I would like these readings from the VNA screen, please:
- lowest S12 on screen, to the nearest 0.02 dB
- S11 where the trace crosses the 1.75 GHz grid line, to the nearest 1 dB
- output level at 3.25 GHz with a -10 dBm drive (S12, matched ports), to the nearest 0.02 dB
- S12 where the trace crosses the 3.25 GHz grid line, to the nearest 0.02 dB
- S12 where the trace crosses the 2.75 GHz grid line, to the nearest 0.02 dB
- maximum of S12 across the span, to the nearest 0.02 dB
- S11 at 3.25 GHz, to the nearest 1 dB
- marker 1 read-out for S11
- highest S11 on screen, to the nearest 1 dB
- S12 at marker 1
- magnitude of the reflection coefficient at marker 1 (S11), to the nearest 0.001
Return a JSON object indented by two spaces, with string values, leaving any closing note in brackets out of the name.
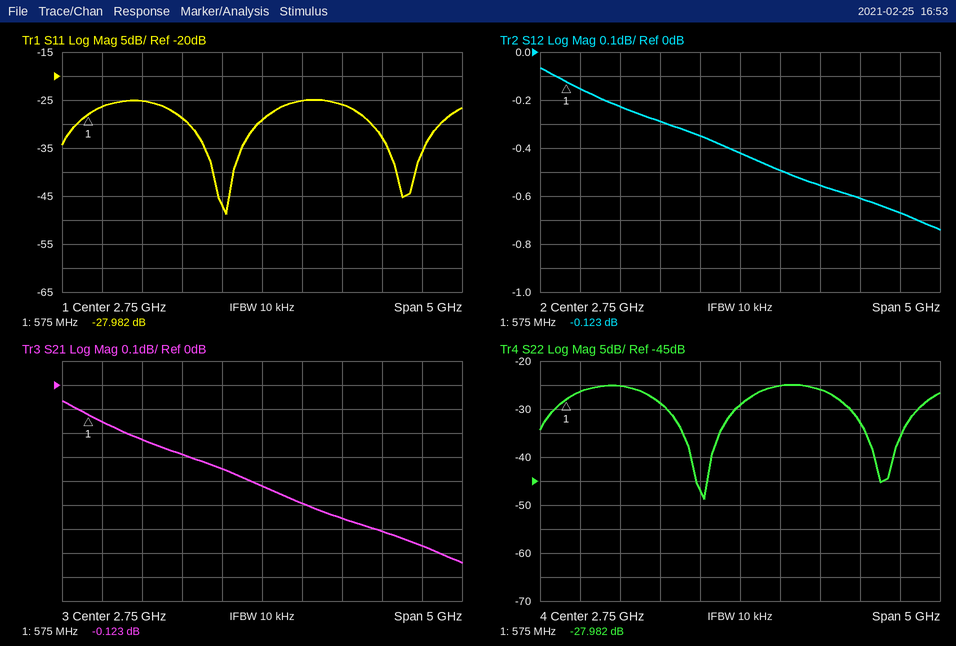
{
  "lowest S12 on screen, to the nearest 0.02 dB": "-0.74 dB",
  "S11 where the trace crosses the 1.75 GHz grid line, to the nearest 1 dB": "-29 dB",
  "output level at 3.25 GHz with a -10 dBm drive (S12, matched ports), to the nearest 0.02 dB": "-10.50 dBm",
  "S12 where the trace crosses the 3.25 GHz grid line, to the nearest 0.02 dB": "-0.50 dB",
  "S12 where the trace crosses the 2.75 GHz grid line, to the nearest 0.02 dB": "-0.42 dB",
  "maximum of S12 across the span, to the nearest 0.02 dB": "-0.06 dB",
  "S11 at 3.25 GHz, to the nearest 1 dB": "-25 dB",
  "marker 1 read-out for S11": "-27.982 dB",
  "highest S11 on screen, to the nearest 1 dB": "-25 dB",
  "S12 at marker 1": "-0.123 dB",
  "magnitude of the reflection coefficient at marker 1 (S11), to the nearest 0.001": "0.040"
}
